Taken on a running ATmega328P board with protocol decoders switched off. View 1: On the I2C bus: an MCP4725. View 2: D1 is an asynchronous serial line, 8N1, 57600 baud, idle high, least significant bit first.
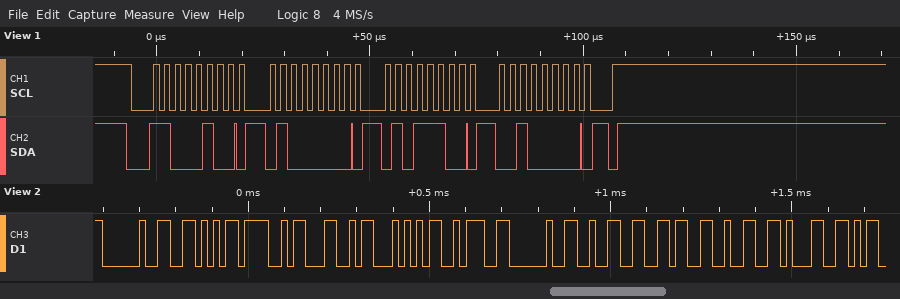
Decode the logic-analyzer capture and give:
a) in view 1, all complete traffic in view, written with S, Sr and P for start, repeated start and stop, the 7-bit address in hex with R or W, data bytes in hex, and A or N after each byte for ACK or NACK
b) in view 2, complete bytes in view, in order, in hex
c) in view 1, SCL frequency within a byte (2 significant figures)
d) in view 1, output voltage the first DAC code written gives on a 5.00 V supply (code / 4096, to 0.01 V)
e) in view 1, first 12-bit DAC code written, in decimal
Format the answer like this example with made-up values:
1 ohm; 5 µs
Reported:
S 62W A 40 A 5C A 20 A P; 20 56 4F 4C 54 3A 20 32 36 32 31; 400 kHz; 1.80 V; 1474
